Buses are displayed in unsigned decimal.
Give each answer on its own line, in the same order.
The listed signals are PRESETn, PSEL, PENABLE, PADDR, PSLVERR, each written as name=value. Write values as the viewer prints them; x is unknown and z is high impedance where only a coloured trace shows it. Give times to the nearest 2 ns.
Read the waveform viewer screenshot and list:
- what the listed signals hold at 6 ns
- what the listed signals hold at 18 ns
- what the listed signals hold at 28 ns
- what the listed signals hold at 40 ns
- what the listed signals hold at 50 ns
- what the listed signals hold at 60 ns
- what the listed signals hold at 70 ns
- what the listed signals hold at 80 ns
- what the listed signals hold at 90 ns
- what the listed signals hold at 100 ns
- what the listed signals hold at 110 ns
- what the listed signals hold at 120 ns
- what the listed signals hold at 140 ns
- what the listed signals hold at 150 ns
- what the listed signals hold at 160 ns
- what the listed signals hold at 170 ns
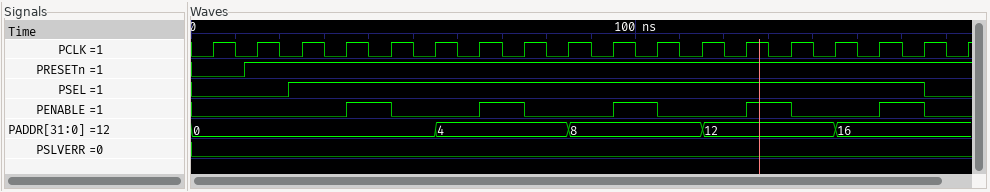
PRESETn=0, PSEL=0, PENABLE=0, PADDR=0, PSLVERR=0
PRESETn=1, PSEL=0, PENABLE=0, PADDR=0, PSLVERR=0
PRESETn=1, PSEL=1, PENABLE=0, PADDR=0, PSLVERR=0
PRESETn=1, PSEL=1, PENABLE=1, PADDR=0, PSLVERR=0
PRESETn=1, PSEL=1, PENABLE=0, PADDR=0, PSLVERR=0
PRESETn=1, PSEL=1, PENABLE=0, PADDR=4, PSLVERR=0
PRESETn=1, PSEL=1, PENABLE=1, PADDR=4, PSLVERR=0
PRESETn=1, PSEL=1, PENABLE=0, PADDR=4, PSLVERR=0
PRESETn=1, PSEL=1, PENABLE=0, PADDR=8, PSLVERR=0
PRESETn=1, PSEL=1, PENABLE=1, PADDR=8, PSLVERR=0
PRESETn=1, PSEL=1, PENABLE=0, PADDR=8, PSLVERR=0
PRESETn=1, PSEL=1, PENABLE=0, PADDR=12, PSLVERR=0
PRESETn=1, PSEL=1, PENABLE=0, PADDR=12, PSLVERR=0
PRESETn=1, PSEL=1, PENABLE=0, PADDR=16, PSLVERR=0
PRESETn=1, PSEL=1, PENABLE=1, PADDR=16, PSLVERR=0
PRESETn=1, PSEL=0, PENABLE=0, PADDR=16, PSLVERR=0
